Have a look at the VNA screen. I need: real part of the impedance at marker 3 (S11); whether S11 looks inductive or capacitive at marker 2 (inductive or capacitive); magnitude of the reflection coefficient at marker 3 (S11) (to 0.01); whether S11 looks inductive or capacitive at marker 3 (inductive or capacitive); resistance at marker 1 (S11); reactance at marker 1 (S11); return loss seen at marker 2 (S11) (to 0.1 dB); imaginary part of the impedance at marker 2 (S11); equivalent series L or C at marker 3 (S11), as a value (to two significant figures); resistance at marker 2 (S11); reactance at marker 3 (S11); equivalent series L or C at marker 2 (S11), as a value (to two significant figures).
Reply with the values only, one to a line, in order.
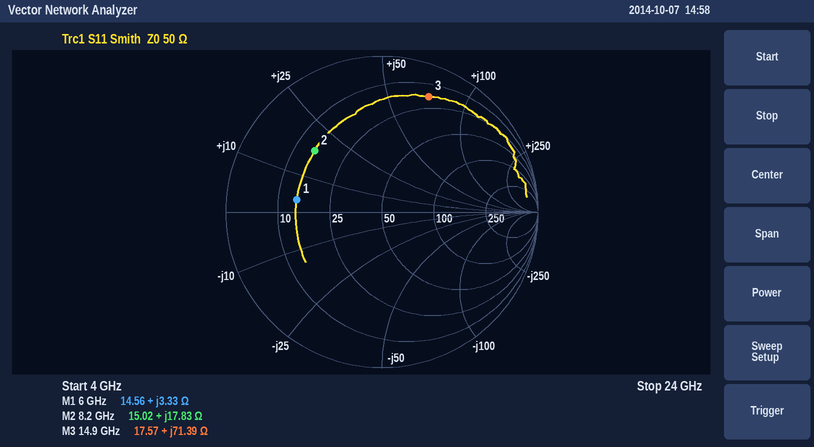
17.57 Ω
inductive
0.80
inductive
14.56 Ω
+3.33 Ω
4.7 dB
+17.83 Ω
760 pH
15.02 Ω
+71.39 Ω
350 pH
